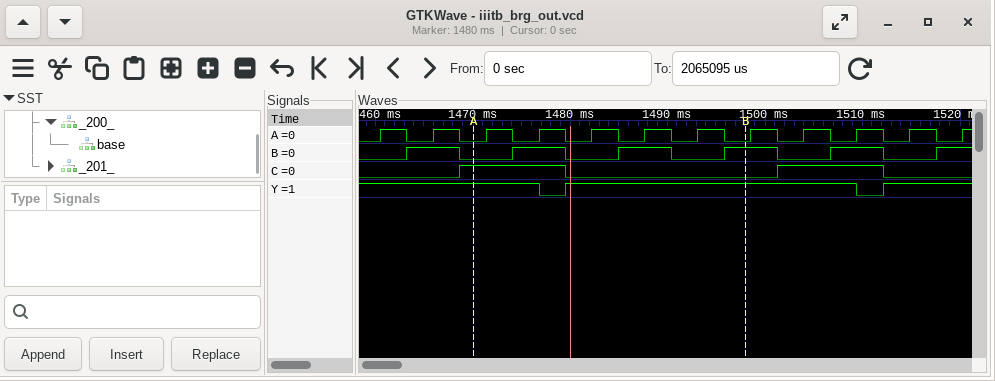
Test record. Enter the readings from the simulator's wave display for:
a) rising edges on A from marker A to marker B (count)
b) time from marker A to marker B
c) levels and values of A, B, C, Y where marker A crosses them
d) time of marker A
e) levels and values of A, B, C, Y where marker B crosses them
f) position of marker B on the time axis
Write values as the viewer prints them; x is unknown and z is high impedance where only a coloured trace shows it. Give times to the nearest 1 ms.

5
28 ms
A=0, B=0, C=1, Y=1
1470 ms
A=0, B=1, C=0, Y=1
1498 ms
